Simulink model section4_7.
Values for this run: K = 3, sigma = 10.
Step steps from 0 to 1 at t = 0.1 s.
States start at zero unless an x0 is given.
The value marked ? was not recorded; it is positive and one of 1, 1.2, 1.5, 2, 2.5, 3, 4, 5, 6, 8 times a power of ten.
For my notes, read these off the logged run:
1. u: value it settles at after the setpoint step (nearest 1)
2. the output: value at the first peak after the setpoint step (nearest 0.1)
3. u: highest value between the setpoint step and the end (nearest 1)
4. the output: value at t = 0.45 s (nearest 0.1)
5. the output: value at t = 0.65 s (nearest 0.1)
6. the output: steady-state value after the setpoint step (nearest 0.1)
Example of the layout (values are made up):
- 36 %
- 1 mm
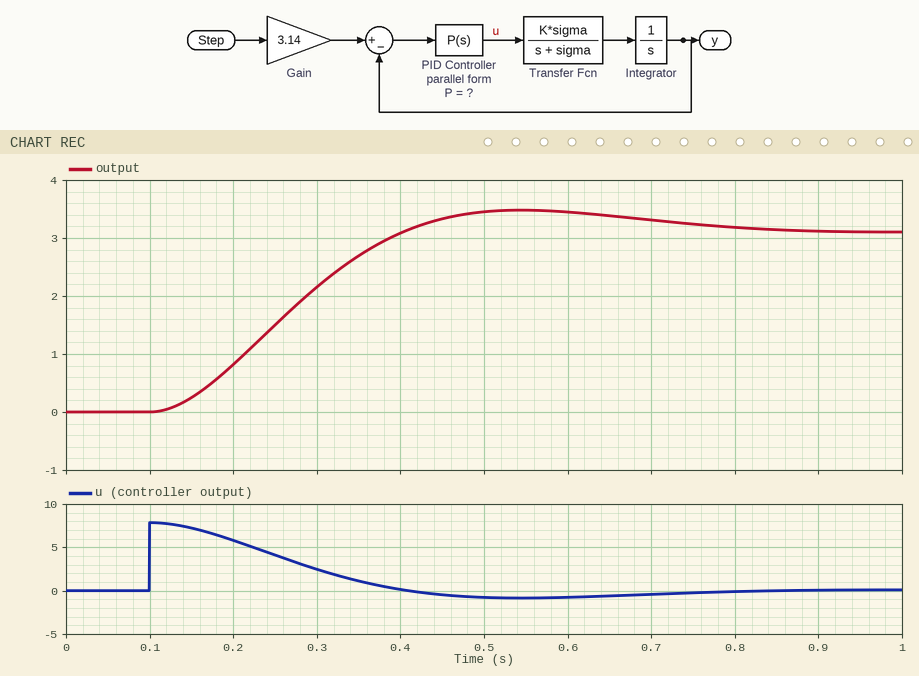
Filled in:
- 0
- 3.5
- 8
- 3.3
- 3.4
- 3.1
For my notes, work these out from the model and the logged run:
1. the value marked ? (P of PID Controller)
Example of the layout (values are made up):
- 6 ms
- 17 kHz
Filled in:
- 2.5
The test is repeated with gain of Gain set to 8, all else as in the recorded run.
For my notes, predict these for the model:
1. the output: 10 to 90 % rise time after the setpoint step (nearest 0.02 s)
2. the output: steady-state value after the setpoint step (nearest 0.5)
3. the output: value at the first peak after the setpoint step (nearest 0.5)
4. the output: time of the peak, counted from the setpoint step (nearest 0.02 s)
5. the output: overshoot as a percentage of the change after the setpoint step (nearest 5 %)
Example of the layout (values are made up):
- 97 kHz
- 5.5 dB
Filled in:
- 0.20 s
- 8.0
- 9.0
- 0.44 s
- 10 %
